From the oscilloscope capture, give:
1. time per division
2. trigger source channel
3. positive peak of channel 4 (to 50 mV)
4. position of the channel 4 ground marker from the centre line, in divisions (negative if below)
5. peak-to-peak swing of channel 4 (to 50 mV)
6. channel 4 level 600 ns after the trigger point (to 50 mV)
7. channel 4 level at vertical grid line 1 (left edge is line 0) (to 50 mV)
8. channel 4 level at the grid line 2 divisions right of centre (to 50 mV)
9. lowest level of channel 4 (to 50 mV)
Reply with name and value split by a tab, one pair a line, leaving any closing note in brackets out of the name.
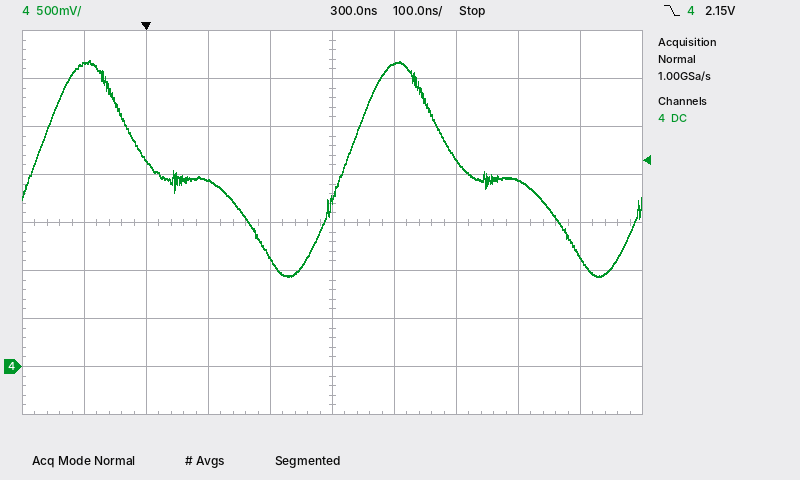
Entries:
time per division	100 ns
trigger source channel	channel 4
positive peak of channel 4	3.20 V
position of the channel 4 ground marker from the centre line, in divisions	-3.0 div
peak-to-peak swing of channel 4	2.25 V
channel 4 level 600 ns after the trigger point	1.95 V
channel 4 level at vertical grid line 1 (left edge is line 0)	3.15 V
channel 4 level at the grid line 2 divisions right of centre	2.15 V
lowest level of channel 4	950 mV
